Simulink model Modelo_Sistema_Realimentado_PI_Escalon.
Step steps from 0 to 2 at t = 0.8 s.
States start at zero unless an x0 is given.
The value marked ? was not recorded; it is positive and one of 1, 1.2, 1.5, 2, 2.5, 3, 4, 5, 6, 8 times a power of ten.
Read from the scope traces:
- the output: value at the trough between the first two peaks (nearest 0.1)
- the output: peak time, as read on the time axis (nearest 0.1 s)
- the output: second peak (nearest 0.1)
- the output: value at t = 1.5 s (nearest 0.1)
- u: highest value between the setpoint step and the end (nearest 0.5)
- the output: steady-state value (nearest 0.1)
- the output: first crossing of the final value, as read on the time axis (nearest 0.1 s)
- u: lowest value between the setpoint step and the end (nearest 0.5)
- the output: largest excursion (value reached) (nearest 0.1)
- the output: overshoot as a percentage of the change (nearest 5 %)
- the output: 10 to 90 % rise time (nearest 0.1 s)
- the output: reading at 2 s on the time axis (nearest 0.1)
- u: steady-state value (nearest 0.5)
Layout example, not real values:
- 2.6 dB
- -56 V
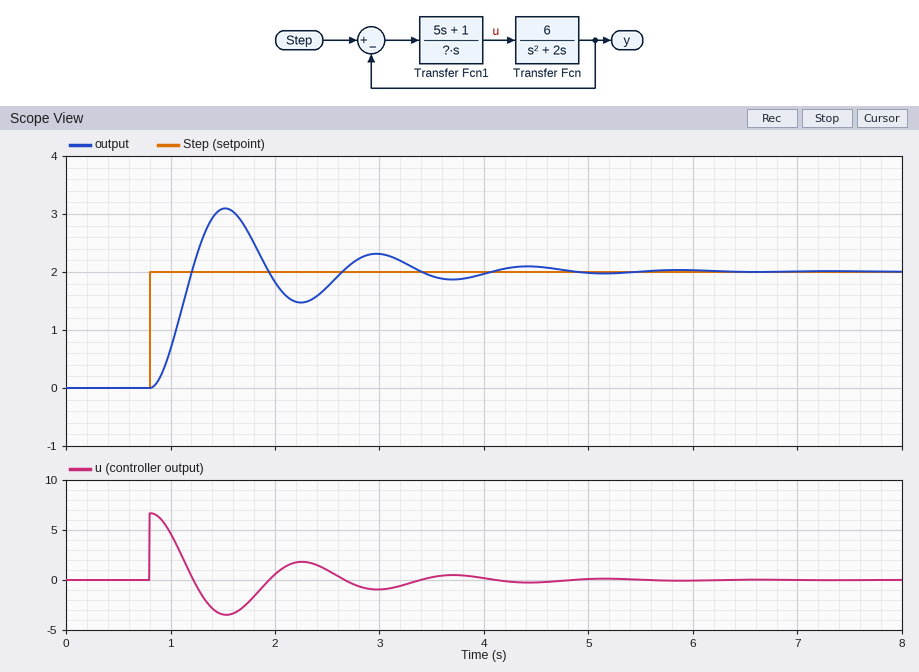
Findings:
- 1.5
- 1.5 s
- 2.3
- 3.1
- 6.5
- 2.0
- 1.2 s
- -3.5
- 3.1
- 55 %
- 0.3 s
- 1.8
- 0.0
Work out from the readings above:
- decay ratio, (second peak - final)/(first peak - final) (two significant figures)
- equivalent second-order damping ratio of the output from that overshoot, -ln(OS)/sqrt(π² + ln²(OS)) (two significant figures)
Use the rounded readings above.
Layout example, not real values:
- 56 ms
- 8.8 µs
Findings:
- 0.27
- 0.19
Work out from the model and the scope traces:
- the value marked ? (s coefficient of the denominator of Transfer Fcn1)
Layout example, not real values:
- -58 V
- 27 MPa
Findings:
- 1.5
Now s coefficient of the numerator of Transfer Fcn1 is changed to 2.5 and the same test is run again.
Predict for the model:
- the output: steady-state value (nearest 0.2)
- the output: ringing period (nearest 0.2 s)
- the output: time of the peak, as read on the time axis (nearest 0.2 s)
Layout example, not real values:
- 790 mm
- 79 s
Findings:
- 2.0
- 2.2 s
- 1.8 s
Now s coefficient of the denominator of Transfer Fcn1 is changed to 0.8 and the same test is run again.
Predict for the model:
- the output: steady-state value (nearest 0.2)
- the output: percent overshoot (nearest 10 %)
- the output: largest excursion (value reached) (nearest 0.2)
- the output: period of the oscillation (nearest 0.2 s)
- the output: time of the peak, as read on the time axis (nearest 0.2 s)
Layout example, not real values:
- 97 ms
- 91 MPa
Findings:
- 2.0
- 60 %
- 3.2
- 1.0 s
- 1.4 s
